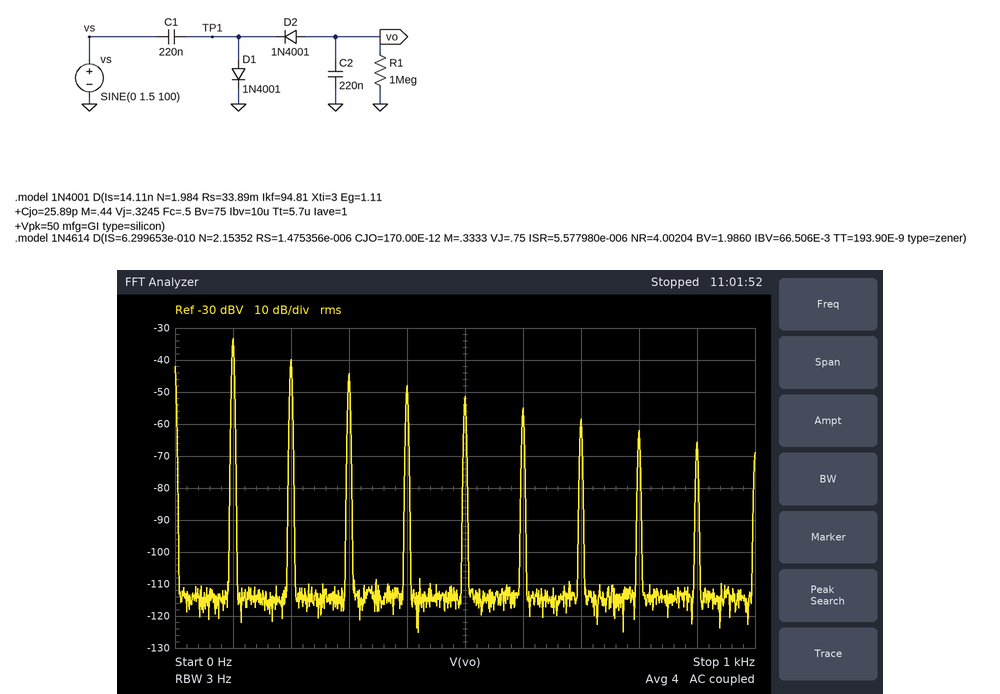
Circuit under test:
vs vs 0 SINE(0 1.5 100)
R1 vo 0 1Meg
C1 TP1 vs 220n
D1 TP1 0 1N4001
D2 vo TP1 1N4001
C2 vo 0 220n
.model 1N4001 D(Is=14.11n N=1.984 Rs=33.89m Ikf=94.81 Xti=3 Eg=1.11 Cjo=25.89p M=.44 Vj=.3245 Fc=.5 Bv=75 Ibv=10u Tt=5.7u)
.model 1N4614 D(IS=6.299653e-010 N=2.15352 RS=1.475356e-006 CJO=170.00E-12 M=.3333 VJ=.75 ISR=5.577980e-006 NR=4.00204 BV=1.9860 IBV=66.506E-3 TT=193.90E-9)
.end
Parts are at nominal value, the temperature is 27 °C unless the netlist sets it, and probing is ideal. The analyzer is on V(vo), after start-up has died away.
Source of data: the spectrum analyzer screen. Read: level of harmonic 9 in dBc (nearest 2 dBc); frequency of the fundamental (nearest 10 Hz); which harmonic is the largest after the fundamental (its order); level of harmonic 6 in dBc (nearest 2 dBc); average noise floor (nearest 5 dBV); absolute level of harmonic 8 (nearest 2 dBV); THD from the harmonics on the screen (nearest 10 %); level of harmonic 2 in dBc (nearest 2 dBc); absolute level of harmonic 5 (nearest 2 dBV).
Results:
-32 dBc
100 Hz
2
-22 dBc
-115 dBV
-62 dBV
60 %
-6 dBc
-52 dBV
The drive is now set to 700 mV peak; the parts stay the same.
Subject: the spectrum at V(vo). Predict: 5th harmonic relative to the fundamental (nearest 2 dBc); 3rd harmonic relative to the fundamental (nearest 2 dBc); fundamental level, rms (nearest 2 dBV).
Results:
-22 dBc
-12 dBc
-42 dBV
